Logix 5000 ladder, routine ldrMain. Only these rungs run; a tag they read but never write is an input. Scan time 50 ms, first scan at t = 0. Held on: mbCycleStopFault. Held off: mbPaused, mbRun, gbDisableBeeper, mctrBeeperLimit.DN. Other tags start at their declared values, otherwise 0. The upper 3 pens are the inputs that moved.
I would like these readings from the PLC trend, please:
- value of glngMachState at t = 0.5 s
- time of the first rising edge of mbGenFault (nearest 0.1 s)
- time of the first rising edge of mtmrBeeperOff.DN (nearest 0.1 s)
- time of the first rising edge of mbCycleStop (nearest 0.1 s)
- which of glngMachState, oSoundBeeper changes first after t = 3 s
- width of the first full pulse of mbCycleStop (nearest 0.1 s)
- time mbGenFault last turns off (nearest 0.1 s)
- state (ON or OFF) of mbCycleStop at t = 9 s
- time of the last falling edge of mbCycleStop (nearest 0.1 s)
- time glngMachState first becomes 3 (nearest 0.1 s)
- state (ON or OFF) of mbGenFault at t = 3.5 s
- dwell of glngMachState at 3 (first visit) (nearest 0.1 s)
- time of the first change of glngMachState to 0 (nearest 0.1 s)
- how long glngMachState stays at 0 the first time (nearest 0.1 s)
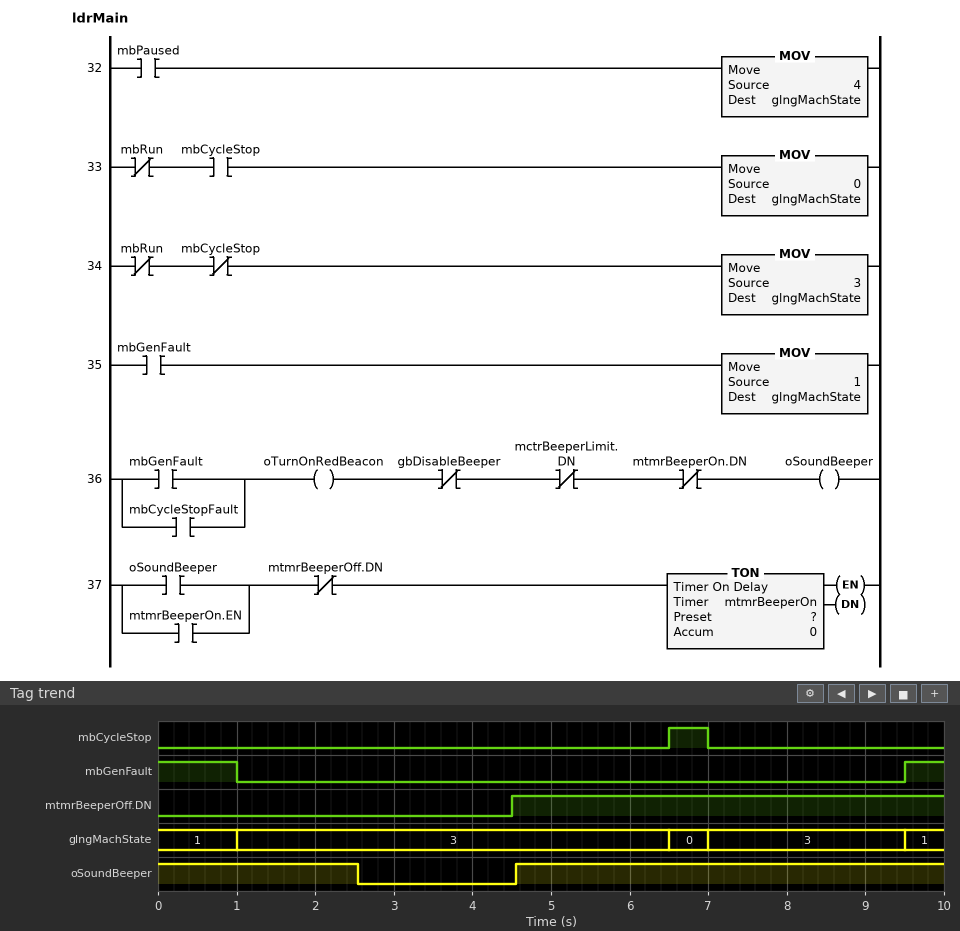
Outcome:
1
9.5 s
4.5 s
6.5 s
oSoundBeeper
0.5 s
1.0 s
OFF
7.0 s
1.0 s
OFF
5.5 s
6.5 s
0.5 s
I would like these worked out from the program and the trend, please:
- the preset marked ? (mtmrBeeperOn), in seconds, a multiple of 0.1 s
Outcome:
2.5 s
